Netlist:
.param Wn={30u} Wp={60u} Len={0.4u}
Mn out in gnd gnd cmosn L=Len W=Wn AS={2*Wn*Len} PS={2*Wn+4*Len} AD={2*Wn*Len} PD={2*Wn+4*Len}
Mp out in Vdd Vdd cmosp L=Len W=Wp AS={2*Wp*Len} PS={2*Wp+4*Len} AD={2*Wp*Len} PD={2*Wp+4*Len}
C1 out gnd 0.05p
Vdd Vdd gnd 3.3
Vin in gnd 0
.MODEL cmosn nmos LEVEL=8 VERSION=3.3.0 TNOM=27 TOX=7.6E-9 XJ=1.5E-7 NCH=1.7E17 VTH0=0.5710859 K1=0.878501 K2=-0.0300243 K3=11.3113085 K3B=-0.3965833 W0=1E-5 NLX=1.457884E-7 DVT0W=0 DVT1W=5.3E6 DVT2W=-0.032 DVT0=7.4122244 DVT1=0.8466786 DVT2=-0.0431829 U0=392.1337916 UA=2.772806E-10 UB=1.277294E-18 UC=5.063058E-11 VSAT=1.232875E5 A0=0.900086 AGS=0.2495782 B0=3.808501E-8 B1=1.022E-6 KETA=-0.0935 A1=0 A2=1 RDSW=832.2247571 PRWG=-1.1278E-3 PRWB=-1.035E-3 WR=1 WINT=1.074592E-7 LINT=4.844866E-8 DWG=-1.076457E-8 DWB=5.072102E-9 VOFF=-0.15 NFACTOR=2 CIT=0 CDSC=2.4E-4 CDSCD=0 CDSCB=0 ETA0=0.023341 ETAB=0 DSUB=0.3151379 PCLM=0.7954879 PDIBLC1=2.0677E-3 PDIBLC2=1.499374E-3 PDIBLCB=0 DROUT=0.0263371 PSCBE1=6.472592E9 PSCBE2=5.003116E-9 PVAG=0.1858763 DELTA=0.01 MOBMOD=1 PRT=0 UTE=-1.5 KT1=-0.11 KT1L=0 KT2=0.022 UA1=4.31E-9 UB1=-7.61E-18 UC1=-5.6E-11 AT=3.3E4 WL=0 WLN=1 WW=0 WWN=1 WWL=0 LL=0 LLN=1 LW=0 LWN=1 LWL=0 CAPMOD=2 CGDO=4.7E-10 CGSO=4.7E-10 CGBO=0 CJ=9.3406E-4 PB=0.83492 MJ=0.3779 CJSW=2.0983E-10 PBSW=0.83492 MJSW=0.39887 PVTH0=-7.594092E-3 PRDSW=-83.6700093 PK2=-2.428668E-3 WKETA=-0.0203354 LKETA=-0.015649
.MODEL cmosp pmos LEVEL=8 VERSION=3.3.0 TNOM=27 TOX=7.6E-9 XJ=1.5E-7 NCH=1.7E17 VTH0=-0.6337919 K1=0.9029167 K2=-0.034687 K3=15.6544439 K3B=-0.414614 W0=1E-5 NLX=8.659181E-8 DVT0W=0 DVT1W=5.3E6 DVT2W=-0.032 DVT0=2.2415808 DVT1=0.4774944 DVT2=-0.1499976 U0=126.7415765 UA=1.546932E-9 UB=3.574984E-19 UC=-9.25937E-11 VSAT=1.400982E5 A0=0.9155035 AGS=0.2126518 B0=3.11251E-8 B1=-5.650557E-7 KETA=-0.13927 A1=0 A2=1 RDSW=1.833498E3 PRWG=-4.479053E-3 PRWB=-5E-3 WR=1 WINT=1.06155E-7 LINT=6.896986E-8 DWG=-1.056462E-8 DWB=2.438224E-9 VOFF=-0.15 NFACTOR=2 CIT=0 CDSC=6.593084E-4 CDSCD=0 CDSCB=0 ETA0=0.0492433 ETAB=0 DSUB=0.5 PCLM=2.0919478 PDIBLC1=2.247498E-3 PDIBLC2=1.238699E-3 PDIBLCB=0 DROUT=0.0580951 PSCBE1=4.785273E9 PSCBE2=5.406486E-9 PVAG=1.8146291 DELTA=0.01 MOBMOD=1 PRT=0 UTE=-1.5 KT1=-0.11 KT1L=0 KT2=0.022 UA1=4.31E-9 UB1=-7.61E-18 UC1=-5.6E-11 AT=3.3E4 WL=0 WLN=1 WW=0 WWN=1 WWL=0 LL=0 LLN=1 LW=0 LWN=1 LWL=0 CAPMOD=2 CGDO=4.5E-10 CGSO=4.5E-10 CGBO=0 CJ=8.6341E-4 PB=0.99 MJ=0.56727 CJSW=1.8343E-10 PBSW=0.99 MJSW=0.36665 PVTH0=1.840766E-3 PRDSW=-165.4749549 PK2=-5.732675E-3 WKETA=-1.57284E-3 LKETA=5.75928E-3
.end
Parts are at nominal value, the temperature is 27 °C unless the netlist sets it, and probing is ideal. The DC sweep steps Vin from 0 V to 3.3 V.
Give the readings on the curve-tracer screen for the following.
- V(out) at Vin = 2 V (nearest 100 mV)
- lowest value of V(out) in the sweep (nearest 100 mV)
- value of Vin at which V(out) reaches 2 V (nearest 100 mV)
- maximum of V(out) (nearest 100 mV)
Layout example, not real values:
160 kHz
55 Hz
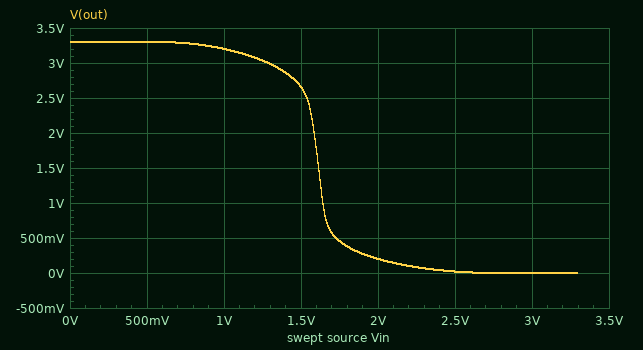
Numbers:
200 mV
0 V
1.6 V
3.3 V
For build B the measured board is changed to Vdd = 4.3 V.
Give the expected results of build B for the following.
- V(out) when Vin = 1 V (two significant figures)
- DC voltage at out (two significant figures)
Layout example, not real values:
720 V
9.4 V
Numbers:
4.2 V
4.3 V
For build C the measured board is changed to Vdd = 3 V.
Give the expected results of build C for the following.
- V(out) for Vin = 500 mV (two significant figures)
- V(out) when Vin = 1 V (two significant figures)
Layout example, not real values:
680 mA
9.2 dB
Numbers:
3.0 V
2.9 V
